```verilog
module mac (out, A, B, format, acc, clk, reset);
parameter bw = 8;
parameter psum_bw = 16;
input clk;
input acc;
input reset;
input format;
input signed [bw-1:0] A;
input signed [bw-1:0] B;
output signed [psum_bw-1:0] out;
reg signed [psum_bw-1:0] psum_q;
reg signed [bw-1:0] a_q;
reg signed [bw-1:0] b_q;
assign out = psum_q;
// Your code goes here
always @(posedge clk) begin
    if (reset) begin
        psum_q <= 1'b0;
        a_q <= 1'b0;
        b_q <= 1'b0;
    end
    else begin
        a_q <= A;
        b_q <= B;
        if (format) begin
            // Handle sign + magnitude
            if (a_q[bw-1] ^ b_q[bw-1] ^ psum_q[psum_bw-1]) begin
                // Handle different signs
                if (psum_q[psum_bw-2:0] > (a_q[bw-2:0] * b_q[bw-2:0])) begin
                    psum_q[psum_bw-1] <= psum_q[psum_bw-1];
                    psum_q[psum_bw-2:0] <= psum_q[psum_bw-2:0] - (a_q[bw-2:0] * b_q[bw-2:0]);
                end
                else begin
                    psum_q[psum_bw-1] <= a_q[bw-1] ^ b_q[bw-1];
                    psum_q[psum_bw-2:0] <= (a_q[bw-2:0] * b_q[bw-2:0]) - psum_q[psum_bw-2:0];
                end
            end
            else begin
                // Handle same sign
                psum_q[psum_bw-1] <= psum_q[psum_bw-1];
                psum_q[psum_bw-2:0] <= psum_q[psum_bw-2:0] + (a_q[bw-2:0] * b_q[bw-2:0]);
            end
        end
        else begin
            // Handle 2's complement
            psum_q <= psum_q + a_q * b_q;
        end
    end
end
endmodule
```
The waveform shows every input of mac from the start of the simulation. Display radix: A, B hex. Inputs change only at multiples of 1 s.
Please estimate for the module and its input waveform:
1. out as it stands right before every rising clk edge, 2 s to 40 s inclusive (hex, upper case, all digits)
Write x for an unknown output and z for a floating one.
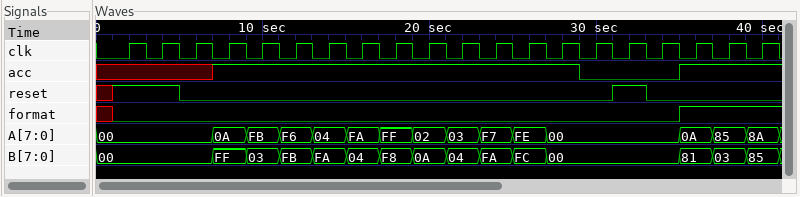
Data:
x, 0000, 0000, 0000, 0000, FFF6, FFE7, 0019, 0001, FFE9, FFF1, 0005, 0011, 0047, 004F, 004F, 0000, 0000, 0000, 800A
